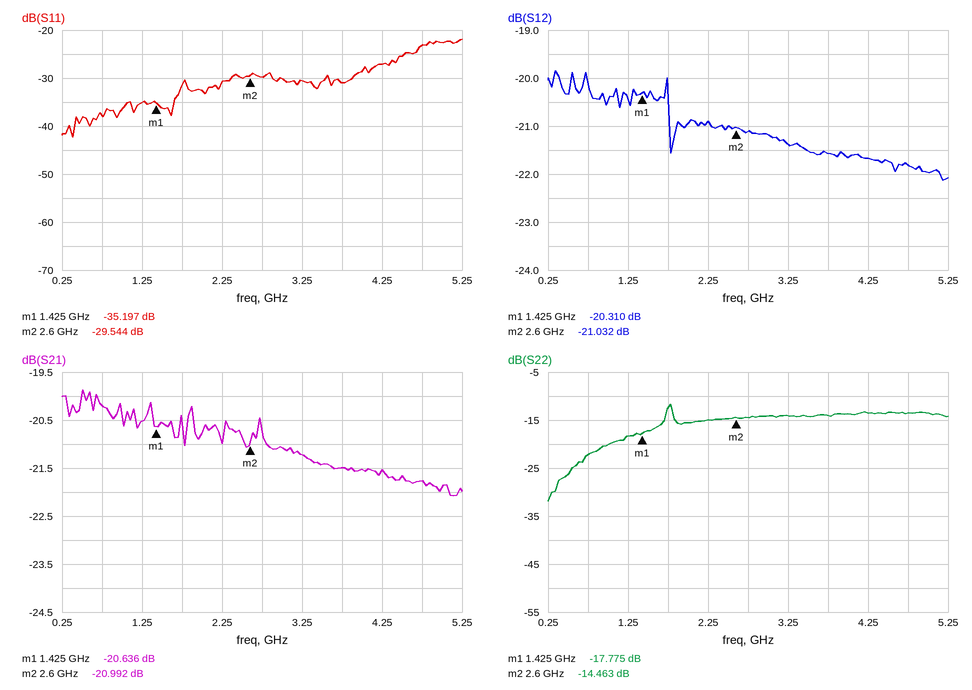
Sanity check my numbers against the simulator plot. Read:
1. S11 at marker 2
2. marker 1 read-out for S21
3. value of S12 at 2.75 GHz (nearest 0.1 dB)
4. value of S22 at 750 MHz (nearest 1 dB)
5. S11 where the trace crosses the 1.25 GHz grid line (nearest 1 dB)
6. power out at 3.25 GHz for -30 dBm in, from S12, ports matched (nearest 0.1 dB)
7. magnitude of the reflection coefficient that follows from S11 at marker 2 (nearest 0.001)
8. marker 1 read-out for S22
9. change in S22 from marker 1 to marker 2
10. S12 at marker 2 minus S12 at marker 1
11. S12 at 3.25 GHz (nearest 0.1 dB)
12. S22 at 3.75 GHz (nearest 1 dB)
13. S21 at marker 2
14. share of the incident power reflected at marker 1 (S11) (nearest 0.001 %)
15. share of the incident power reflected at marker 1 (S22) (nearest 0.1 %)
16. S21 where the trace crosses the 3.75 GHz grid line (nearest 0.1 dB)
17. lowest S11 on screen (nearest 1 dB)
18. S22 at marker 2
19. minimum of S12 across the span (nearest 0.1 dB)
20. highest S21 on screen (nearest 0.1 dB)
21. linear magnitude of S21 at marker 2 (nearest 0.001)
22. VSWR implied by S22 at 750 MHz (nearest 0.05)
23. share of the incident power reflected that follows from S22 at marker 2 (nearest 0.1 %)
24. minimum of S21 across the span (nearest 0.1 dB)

-29.544 dB
-20.636 dB
-21.1 dB
-22 dB
-35 dB
-51.4 dBm
0.033
-17.775 dB
3.312 dB
-0.722 dB
-21.4 dB
-14 dB
-20.992 dB
0.030 %
1.7 %
-21.5 dB
-42 dB
-14.463 dB
-22.1 dB
-19.9 dB
0.089
1.15
3.6 %
-22.1 dB
